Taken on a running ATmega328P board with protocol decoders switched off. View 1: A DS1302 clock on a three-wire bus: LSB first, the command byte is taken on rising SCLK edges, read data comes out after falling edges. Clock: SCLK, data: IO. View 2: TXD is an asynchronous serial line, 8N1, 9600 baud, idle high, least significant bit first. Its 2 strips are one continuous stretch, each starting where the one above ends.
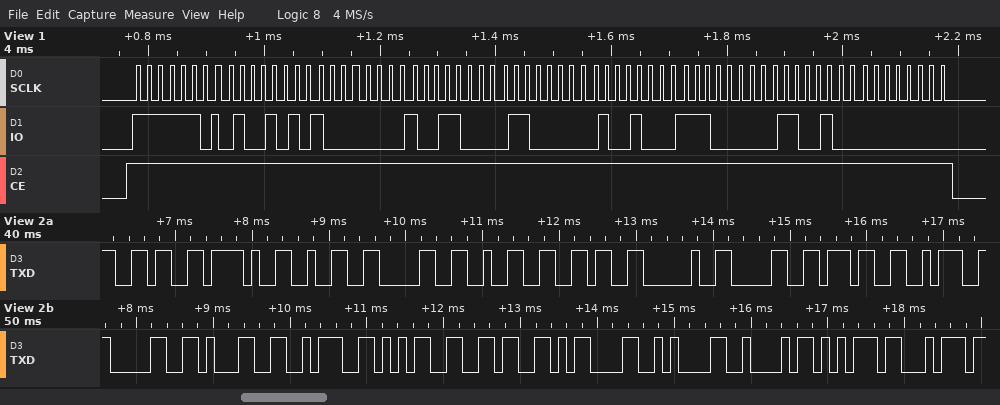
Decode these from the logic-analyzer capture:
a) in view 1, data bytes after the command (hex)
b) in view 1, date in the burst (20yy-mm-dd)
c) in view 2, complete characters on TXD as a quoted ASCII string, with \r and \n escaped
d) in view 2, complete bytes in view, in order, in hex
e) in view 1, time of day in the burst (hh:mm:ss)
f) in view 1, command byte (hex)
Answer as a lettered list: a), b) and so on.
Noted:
a) 52 01 19 06 12 07 26 00
b) 2026-12-06
c) "6/2026 07:01:56\r\nBut"
d) 36 2F 32 30 32 36 20 30 37 3A 30 31 3A 35 36 0D 0A 42 75 74
e) 19:01:52
f) 0xBF
